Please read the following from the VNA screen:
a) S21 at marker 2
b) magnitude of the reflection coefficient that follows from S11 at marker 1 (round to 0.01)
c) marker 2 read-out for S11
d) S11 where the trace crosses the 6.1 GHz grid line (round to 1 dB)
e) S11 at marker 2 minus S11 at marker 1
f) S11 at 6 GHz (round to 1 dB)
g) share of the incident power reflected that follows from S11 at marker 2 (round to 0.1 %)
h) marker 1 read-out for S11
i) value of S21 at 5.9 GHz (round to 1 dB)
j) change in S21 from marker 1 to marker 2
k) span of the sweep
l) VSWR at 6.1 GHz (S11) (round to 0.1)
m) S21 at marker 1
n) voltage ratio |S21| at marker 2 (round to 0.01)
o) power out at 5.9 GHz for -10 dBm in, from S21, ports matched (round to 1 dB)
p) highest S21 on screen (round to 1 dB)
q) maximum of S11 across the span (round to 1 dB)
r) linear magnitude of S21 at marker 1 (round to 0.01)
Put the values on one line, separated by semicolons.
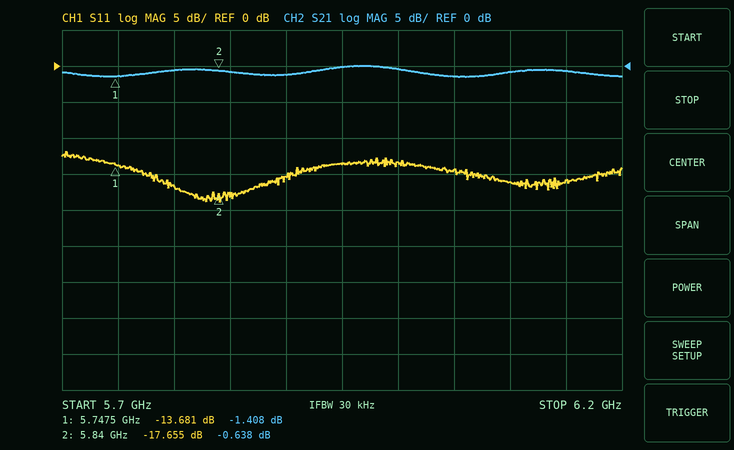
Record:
-0.638 dB; 0.21; -17.655 dB; -16 dB; -3.974 dB; -13 dB; 1.7 %; -13.681 dB; -1 dB; 0.770 dB; 500 MHz; 1.4; -1.408 dB; 0.93; -11 dBm; 0 dB; -12 dB; 0.85
